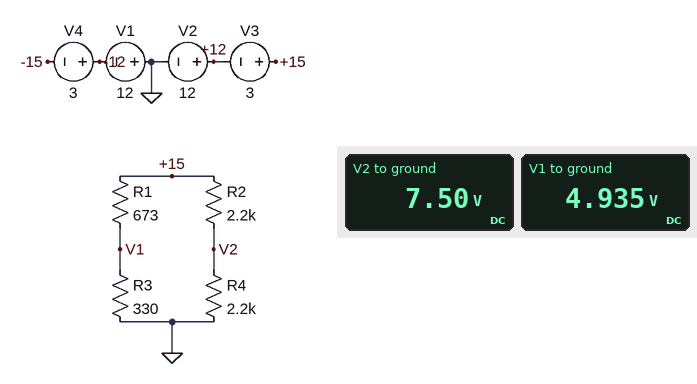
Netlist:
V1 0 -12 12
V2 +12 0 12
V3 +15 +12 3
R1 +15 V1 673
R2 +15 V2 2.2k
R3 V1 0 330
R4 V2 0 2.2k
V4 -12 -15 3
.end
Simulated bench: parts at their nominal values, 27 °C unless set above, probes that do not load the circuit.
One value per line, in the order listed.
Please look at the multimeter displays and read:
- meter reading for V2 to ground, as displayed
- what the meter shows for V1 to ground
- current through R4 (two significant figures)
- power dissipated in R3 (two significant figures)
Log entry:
7.50 V
4.935 V
3.4 mA
74 mW
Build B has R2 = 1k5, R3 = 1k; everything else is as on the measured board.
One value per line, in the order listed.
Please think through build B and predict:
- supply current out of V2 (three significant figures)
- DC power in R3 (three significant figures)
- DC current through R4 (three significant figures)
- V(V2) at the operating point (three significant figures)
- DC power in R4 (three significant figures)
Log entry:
13.0 mA
80.4 mW
4.05 mA
8.92 V
36.2 mW
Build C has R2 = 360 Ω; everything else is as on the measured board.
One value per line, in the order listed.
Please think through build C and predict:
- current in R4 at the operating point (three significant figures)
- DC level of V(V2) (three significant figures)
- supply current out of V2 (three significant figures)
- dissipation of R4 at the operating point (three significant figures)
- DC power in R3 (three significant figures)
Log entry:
5.86 mA
12.9 V
20.8 mA
75.5 mW
73.8 mW
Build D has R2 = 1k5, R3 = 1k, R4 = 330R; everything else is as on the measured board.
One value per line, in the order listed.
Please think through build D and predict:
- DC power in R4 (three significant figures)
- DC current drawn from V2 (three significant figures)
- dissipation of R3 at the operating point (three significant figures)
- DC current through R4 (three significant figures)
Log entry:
22.2 mW
17.2 mA
80.4 mW
8.20 mA
